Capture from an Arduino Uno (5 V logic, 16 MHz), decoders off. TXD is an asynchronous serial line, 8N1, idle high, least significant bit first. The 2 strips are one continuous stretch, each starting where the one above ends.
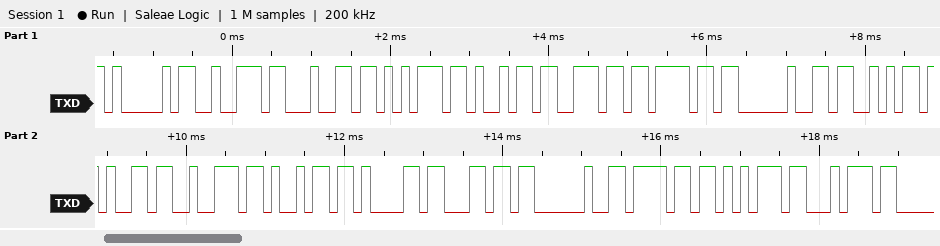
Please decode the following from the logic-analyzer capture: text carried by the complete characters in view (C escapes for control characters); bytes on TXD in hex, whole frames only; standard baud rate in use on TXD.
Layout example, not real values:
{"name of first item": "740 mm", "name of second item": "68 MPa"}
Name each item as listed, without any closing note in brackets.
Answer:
{"text carried by the complete characters in view": "\"Arduino Serial out\"", "bytes on TXD in hex, whole frames only": "41 72 64 75 69 6E 6F 20 53 65 72 69 61 6C 20 6F 75 74", "standard baud rate in use on TXD": "9600 baud"}
